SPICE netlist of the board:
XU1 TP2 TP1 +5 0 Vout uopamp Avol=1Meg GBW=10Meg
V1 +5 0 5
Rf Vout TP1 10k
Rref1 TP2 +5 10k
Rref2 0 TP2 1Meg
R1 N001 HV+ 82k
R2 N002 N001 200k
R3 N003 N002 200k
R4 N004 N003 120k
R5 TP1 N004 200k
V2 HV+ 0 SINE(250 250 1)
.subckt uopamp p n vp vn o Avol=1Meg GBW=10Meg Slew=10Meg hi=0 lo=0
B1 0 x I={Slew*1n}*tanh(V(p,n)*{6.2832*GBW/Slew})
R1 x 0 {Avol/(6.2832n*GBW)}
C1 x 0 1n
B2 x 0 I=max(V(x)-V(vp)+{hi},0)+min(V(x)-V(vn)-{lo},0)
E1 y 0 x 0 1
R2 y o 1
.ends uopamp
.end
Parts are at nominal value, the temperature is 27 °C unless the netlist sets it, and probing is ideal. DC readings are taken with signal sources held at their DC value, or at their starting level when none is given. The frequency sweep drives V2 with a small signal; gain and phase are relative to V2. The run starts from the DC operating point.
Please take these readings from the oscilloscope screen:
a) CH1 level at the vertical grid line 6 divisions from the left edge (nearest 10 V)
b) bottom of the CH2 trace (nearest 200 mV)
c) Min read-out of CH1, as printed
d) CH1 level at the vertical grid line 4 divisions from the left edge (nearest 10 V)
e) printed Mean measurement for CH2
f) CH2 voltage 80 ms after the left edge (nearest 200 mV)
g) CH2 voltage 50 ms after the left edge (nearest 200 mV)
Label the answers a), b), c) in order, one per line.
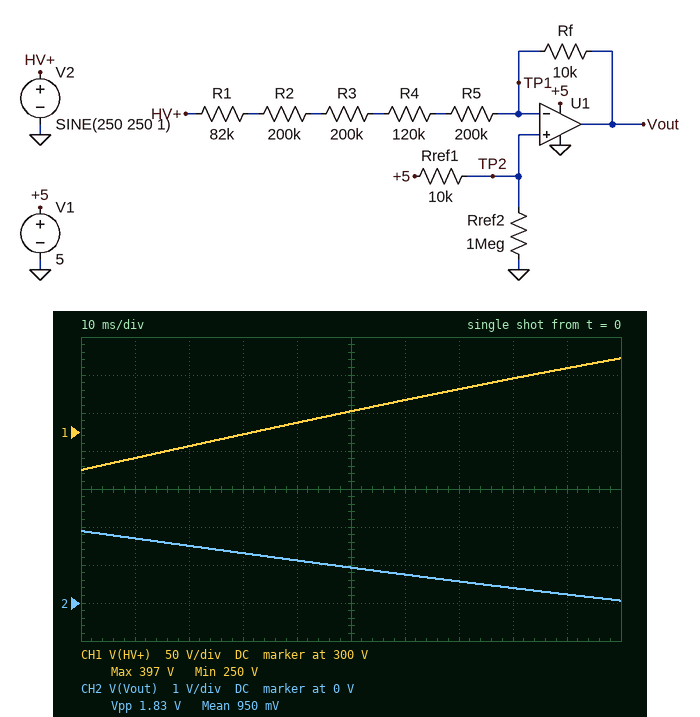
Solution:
a) 340 V
b) 0 V
c) 250 V
d) 310 V
e) 950 mV
f) 400 mV
g) 1.0 V
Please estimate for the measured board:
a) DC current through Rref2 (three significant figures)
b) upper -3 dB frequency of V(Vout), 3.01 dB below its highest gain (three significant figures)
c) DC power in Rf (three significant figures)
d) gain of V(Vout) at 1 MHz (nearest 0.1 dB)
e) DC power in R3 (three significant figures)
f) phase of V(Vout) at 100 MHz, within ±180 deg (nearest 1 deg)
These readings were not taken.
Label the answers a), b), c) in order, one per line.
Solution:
a) 4.95 µA
b) 9.88 MHz
c) 934 µW
d) -38.1 dB
e) 18.7 mW
f) 96 deg
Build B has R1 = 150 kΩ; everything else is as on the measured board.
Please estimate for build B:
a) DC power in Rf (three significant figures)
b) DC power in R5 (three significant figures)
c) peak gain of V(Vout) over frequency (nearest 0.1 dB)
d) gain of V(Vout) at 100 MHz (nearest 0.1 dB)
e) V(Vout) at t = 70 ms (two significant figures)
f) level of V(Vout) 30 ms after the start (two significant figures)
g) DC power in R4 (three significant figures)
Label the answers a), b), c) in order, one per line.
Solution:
a) 793 µW
b) 15.9 mW
c) -38.8 dB
d) -58.9 dB
e) 910 mV
f) 1.6 V
g) 9.52 mW
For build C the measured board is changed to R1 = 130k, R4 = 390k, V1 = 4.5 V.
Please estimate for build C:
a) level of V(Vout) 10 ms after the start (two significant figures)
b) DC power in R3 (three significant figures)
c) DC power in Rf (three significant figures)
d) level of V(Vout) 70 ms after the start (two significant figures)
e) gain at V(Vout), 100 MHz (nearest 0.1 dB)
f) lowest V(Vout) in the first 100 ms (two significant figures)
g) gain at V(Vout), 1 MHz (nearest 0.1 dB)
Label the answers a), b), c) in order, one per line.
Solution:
a) 2.1 V
b) 9.61 mW
c) 481 µW
d) 1.3 V
e) -61.1 dB
f) 950 mV
g) -41.0 dB
